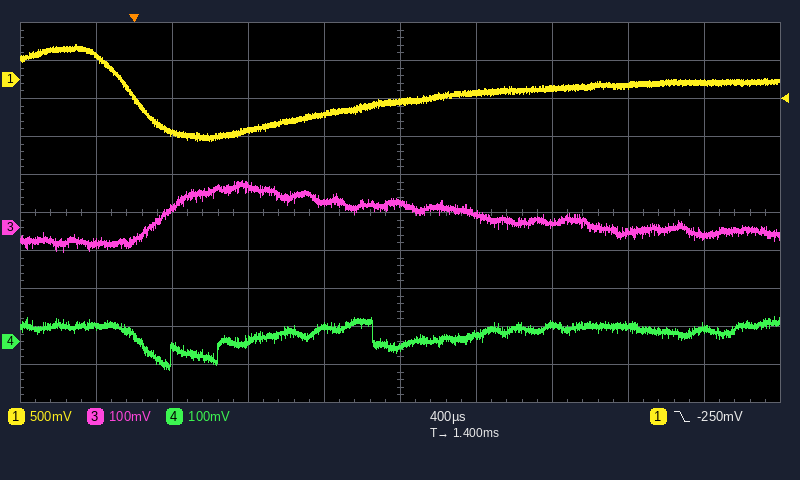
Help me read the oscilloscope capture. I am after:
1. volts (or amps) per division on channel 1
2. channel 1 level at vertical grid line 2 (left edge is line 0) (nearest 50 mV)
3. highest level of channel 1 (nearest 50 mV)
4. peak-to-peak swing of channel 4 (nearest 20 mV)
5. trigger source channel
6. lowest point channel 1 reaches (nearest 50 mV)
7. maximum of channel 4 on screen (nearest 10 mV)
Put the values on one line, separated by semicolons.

500 mV; -700 mV; 450 mV; 140 mV; channel 1; -800 mV; 70 mV
